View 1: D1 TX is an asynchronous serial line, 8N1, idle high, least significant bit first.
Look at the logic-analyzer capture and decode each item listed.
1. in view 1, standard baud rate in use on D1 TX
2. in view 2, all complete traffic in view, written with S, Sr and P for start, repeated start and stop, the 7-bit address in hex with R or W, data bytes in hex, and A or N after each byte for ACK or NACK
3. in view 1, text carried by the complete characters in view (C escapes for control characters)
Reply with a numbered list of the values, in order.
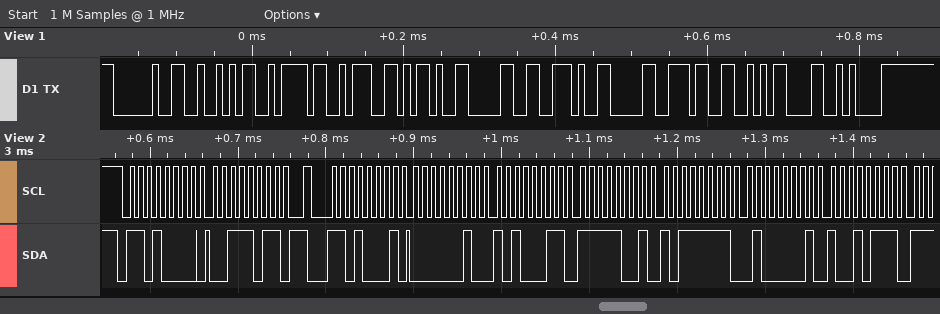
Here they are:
1. 115200 baud
2. S 68W A 3B A Sr 68R A 02 A A3 A F9 A BF A 41 A 97 A
3. " Rz:-0.03\r\n"
